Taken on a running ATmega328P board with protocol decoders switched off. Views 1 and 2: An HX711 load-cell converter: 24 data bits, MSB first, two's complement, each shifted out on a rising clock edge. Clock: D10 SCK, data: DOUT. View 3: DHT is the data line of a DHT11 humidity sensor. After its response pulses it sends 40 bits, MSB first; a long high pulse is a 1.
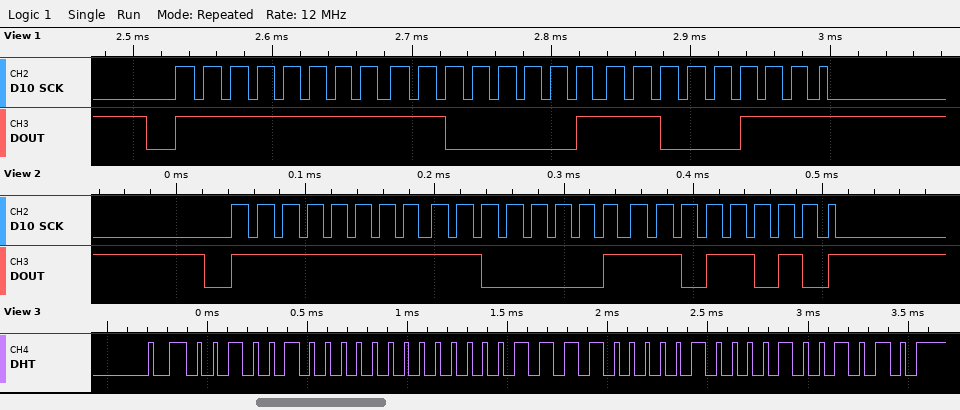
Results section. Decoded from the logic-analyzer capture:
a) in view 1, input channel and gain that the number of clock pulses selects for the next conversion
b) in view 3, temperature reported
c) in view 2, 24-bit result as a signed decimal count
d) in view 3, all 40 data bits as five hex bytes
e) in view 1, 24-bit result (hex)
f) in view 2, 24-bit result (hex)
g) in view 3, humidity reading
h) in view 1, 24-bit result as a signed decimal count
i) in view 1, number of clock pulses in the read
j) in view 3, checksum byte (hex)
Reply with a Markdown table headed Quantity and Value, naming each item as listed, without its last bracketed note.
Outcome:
| Quantity | Value |
|---|---|
| in view 1, input channel and gain that the number of clock pulses selects for the next conversion | channel A, gain 128 |
| in view 3, temperature reported | 30.8 °C |
| in view 2, 24-bit result as a signed decimal count | -15910 |
| in view 3, all 40 data bits as five hex bytes | 24 00 1E 08 4A |
| in view 1, 24-bit result | 0xFFC1C7 |
| in view 2, 24-bit result | 0xFFC1DA |
| in view 3, humidity reading | 36 % |
| in view 1, 24-bit result as a signed decimal count | -15929 |
| in view 1, number of clock pulses in the read | 25 |
| in view 3, checksum byte | 0x4A |
